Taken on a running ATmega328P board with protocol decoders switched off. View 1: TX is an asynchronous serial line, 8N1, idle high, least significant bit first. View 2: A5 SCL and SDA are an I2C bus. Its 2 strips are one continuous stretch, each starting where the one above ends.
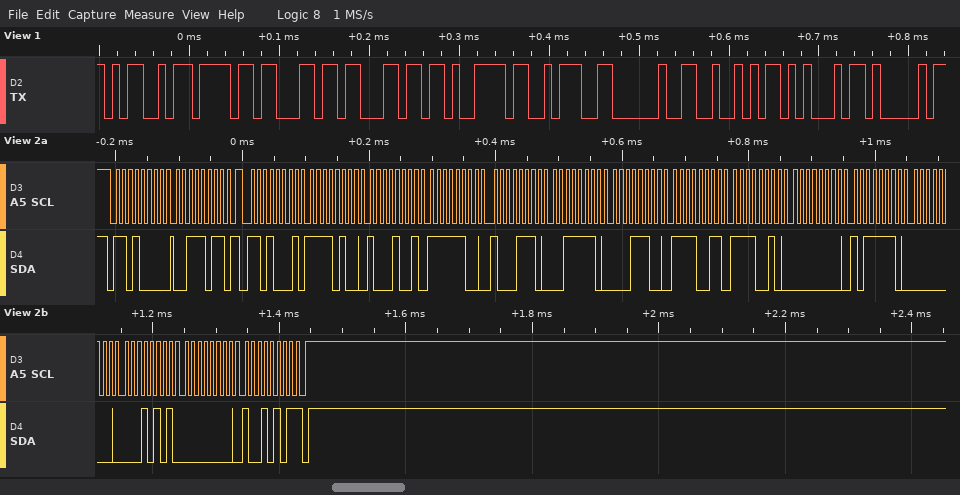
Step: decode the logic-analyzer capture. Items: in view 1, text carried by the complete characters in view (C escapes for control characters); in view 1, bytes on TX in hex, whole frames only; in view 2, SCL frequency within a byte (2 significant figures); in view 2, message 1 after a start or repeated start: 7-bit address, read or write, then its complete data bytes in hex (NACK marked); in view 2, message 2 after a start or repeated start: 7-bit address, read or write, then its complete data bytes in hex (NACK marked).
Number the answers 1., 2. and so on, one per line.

1. "Molly: REA"
2. 0x4D 0x6F 0x6C 0x6C 0x79 0x3A 0x20 0x52 0x45 0x41
3. 100 kHz
4. 0x68 write: 3B
5. 0x68 read: F4 89 FC 8E 3E 1C F3 F2 00 BE 00 15 00 95 NACK
